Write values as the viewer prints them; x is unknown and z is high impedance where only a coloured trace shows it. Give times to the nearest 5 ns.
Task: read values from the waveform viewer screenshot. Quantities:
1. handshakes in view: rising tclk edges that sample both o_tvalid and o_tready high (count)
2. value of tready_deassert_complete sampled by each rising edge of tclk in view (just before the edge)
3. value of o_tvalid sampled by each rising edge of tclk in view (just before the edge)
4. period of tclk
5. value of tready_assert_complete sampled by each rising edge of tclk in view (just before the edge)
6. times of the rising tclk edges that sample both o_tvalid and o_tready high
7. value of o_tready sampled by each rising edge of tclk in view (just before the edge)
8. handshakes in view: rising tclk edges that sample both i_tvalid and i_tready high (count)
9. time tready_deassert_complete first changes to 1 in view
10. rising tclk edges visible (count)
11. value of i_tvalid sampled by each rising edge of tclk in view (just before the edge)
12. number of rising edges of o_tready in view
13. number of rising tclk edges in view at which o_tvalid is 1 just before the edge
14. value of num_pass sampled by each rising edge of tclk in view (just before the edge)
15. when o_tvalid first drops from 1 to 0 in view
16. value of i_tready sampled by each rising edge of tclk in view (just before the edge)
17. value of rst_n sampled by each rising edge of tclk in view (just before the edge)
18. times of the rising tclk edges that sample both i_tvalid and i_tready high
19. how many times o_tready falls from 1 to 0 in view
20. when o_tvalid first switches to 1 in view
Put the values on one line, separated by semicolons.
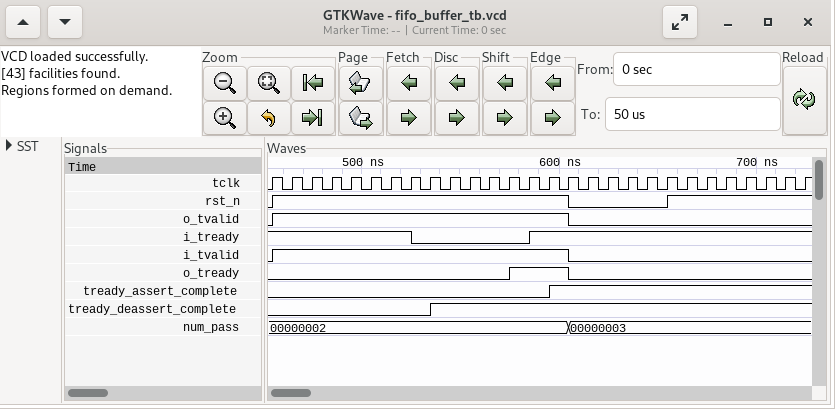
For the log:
3; 0 0 0 0 0 0 0 0 0 1 1 1 1 1 1 1 1 1 1 1 1 1 1 1 1 1 1 1; 0 1 1 1 1 1 1 1 1 1 1 1 1 1 1 1 0 0 0 0 0 0 0 0 0 0 0 0; 10 ns; 0 0 0 0 0 0 0 0 0 0 0 0 0 0 0 1 1 1 1 1 1 1 1 1 1 1 1 1; 585 ns, 595 ns, 605 ns; 0 0 0 0 0 0 0 0 0 0 0 0 0 1 1 1 0 0 0 0 0 0 0 0 0 0 0 0; 9; 535 ns; 28; 0 1 1 1 1 1 1 1 1 1 1 1 1 1 1 1 0 0 0 0 0 0 0 0 0 0 0 0; 1; 15; 00000002, 00000002, 00000002, 00000002, 00000002, 00000002, 00000002, 00000002, 00000002, 00000002, 00000002, 00000002, 00000002, 00000002, 00000002, 00000002, 00000003, 00000003, 00000003, 00000003, 00000003, 00000003, 00000003, 00000003, 00000003, 00000003, 00000003, 00000003; 605 ns; 1 1 1 1 1 1 1 1 0 0 0 0 0 0 1 1 1 1 1 1 1 1 1 1 1 1 1 1; 0 1 1 1 1 1 1 1 1 1 1 1 1 1 1 1 0 0 0 0 0 1 1 1 1 1 1 1; 465 ns, 475 ns, 485 ns, 495 ns, 505 ns, 515 ns, 525 ns, 595 ns, 605 ns; 1; 455 ns
